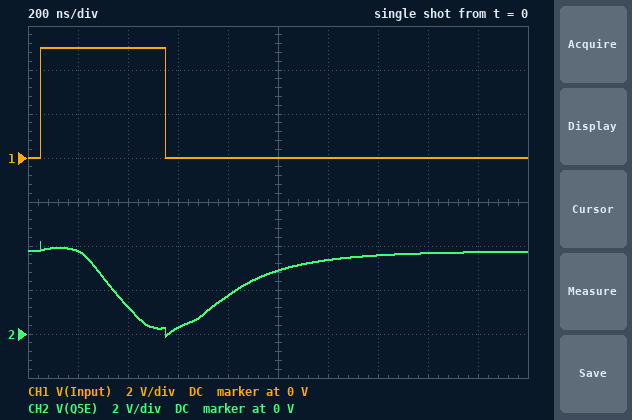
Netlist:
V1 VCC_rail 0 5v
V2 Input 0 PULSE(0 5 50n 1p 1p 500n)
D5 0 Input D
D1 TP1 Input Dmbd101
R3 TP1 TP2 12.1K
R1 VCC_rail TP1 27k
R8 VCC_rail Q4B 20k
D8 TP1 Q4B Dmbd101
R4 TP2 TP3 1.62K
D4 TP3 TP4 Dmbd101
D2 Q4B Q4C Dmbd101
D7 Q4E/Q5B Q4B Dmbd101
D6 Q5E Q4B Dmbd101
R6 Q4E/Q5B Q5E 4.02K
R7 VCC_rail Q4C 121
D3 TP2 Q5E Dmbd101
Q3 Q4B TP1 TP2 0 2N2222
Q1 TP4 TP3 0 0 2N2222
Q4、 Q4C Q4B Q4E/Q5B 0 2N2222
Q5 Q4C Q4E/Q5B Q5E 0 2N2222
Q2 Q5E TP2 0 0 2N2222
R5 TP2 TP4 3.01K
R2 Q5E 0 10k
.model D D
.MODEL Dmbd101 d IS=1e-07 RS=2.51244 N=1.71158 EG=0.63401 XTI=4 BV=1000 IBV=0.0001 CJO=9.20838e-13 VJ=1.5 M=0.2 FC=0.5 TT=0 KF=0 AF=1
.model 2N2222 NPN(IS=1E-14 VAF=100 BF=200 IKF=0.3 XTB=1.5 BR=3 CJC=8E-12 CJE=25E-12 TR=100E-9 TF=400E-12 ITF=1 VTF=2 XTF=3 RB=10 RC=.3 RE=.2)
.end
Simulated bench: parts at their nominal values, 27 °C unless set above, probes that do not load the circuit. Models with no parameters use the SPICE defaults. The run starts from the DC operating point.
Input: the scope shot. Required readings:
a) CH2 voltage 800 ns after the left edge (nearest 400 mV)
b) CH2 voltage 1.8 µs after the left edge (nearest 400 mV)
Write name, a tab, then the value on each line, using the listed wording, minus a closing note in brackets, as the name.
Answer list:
CH2 voltage 800 ns after the left edge	1.6 V
CH2 voltage 1.8 µs after the left edge	3.6 V
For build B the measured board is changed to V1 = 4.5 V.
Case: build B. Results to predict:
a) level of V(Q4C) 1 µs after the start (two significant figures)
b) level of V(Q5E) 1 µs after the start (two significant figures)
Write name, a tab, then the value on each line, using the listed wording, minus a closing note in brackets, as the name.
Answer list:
level of V(Q4C) 1 µs after the start	4.5 V
level of V(Q5E) 1 µs after the start	2.7 V
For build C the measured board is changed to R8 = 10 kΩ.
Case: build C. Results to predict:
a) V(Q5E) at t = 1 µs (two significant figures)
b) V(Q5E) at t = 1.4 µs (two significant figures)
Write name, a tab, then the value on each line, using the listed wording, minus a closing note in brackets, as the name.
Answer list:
V(Q5E) at t = 1 µs	3.6 V
V(Q5E) at t = 1.4 µs	3.8 V
